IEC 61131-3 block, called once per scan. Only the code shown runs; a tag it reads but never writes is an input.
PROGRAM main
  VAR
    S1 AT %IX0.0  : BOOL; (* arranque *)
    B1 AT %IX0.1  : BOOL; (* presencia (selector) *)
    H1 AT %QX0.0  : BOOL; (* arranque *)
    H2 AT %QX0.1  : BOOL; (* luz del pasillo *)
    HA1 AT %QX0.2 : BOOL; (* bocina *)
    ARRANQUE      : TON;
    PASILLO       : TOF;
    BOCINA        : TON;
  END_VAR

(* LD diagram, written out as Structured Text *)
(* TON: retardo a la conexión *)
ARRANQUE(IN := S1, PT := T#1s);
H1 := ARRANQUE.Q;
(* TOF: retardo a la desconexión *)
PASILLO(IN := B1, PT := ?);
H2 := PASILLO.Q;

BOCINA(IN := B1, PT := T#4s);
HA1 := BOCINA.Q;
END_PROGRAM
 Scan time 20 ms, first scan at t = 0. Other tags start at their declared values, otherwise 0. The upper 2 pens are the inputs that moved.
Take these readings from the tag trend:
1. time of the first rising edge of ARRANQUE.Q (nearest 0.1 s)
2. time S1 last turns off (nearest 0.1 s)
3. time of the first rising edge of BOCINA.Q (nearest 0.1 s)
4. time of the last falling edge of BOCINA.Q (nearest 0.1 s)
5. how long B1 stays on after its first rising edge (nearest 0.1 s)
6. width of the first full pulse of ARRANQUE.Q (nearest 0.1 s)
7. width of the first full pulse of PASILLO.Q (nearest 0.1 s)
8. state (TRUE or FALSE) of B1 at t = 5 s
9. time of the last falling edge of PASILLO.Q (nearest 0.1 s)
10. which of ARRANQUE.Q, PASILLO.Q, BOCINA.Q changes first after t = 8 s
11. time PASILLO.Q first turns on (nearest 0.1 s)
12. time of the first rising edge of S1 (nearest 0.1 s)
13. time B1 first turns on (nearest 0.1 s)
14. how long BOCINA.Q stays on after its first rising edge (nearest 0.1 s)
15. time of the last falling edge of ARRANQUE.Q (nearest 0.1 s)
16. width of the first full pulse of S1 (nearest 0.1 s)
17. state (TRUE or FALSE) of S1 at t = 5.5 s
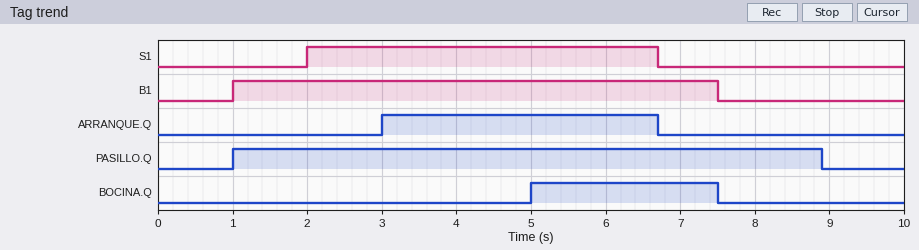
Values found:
3.0 s
6.7 s
5.0 s
7.5 s
6.5 s
3.7 s
7.9 s
TRUE
8.9 s
PASILLO.Q
1.0 s
2.0 s
1.0 s
2.5 s
6.7 s
4.7 s
TRUE
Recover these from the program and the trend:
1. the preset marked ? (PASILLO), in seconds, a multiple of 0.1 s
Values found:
1.4 s
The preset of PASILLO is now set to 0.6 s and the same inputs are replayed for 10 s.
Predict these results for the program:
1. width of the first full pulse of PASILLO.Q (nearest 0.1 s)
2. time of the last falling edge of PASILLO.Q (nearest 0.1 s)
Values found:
7.1 s
8.1 s
